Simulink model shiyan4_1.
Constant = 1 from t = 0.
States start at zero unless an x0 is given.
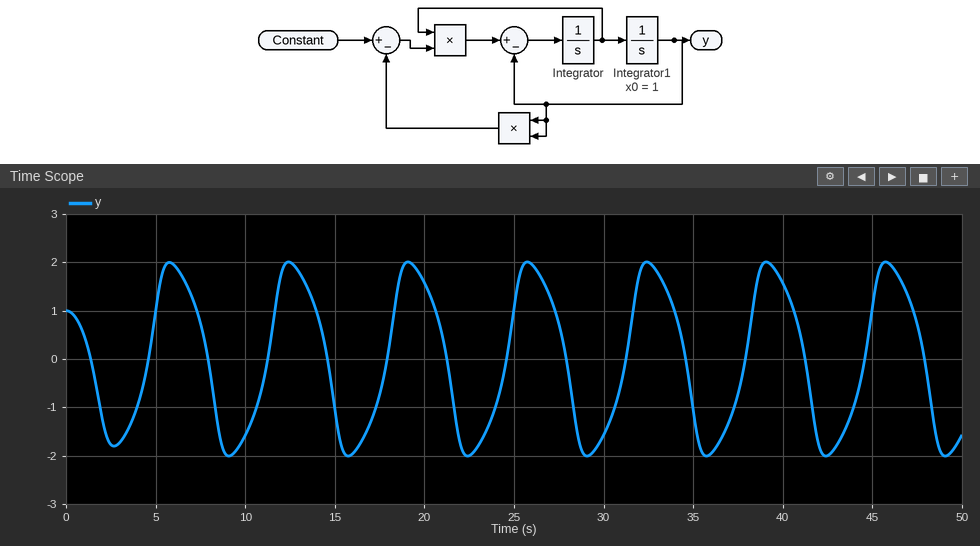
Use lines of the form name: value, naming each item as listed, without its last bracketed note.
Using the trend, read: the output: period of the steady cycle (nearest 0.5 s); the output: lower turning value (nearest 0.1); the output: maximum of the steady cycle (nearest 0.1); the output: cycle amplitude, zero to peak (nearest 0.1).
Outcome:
the output: period of the steady cycle: 6.5 s
the output: lower turning value: -2.0
the output: maximum of the steady cycle: 2.0
the output: cycle amplitude, zero to peak: 2.0
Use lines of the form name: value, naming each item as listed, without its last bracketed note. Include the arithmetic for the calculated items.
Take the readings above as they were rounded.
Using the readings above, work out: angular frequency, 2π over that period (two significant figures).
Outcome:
angular frequency, 2π over that period: 2π / 6.5 = 0.97 rad/s
